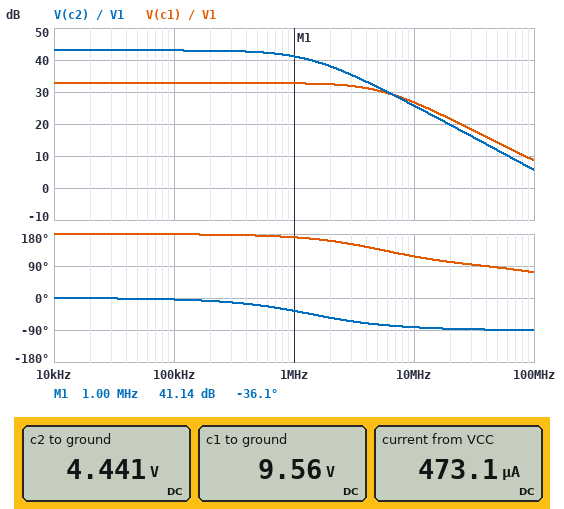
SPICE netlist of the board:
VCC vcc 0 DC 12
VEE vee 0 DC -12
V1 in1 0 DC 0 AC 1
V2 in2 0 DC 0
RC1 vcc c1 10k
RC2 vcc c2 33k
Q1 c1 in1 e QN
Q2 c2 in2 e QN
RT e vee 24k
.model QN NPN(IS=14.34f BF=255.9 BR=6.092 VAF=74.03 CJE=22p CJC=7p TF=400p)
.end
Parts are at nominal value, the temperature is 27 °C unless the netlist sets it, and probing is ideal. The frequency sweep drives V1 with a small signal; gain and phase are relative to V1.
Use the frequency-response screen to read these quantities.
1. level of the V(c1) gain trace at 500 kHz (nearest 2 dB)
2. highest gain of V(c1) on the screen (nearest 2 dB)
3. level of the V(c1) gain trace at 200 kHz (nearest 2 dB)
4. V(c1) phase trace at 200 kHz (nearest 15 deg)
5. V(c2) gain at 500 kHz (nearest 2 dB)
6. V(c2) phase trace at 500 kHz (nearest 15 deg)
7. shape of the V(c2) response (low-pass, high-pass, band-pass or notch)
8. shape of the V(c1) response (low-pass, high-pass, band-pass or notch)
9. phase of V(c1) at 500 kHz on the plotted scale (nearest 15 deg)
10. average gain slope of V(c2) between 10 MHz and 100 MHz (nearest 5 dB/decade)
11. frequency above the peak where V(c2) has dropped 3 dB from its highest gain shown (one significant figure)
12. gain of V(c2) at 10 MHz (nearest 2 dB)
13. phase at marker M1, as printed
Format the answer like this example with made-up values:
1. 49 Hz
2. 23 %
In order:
1. 32 dB
2. 32 dB
3. 32 dB
4. 180 deg
5. 42 dB
6. -15 deg
7. low-pass
8. low-pass
9. 180 deg
10. -20 dB/decade
11. 1 MHz
12. 26 dB
13. -36.1 deg
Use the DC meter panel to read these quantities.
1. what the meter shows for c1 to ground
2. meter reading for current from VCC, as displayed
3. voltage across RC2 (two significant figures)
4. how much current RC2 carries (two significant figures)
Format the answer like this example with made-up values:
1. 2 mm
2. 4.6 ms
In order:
1. 9.56 V
2. 473.1 µA
3. 7.6 V
4. 230 µA
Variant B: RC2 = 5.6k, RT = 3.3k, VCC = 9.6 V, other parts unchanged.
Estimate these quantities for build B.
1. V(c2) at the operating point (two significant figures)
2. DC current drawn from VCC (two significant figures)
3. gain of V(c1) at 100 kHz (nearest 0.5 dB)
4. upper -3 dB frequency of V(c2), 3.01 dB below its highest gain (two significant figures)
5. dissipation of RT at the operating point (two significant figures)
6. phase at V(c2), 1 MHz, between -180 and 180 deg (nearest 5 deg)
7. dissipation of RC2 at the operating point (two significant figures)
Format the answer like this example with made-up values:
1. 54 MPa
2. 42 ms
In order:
1. -650 mV
2. 2.9 mA
3. -11.5 dB
4. 880 MHz
5. 39 mW
6. 0 deg
7. 19 mW
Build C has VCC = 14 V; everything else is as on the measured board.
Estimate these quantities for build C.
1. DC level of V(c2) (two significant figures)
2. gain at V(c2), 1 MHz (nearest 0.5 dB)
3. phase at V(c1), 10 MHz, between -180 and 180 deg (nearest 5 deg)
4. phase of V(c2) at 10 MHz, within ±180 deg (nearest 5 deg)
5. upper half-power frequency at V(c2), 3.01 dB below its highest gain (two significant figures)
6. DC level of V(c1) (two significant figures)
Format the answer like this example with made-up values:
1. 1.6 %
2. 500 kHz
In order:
1. 6.4 V
2. 41.5 dB
3. 120 deg
4. -80 deg
5. 1.5 MHz
6. 12 V
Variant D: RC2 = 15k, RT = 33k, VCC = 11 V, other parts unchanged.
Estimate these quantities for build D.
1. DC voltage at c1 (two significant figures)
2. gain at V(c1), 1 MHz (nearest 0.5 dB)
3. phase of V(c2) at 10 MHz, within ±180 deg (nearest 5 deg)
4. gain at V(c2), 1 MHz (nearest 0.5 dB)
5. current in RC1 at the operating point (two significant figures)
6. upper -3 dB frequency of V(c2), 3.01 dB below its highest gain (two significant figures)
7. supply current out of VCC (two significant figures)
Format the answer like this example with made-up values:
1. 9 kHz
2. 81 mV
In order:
1. 9.3 V
2. 30.0 dB
3. -70 deg
4. 33.5 dB
5. 170 µA
6. 3.5 MHz
7. 340 µA
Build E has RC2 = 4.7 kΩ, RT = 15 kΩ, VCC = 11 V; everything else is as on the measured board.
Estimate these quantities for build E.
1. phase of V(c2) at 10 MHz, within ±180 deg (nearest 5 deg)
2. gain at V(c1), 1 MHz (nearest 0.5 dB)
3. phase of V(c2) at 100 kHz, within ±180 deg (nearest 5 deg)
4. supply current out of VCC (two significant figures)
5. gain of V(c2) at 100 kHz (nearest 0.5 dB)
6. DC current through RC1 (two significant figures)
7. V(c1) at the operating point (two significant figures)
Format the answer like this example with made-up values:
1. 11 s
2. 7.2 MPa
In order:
1. -40 deg
2. 37.0 dB
3. 0 deg
4. 760 µA
5. 30.5 dB
6. 370 µA
7. 7.3 V
